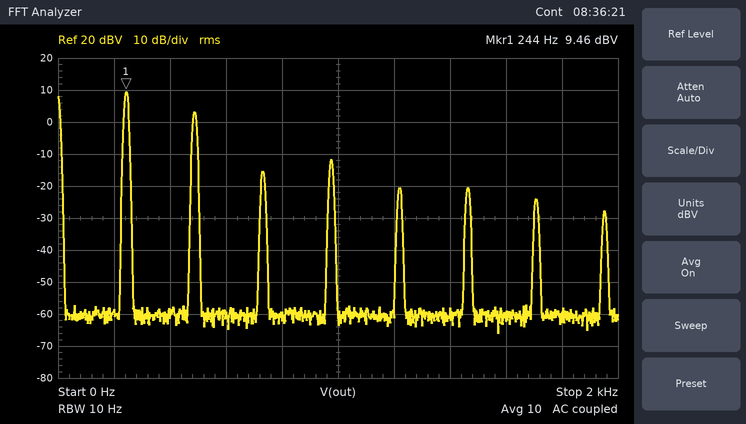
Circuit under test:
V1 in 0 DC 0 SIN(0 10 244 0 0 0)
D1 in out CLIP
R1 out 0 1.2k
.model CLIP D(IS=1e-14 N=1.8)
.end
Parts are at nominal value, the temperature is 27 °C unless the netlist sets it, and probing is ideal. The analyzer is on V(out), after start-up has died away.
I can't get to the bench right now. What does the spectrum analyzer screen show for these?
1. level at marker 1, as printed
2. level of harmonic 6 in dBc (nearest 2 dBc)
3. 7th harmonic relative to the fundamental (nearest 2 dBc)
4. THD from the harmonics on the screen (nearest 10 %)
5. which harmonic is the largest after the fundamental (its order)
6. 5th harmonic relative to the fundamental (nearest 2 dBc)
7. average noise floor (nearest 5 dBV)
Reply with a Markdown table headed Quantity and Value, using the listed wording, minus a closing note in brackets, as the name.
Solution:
| Quantity | Value |
|---|---|
| level at marker 1, as printed | 9.46 dBV |
| level of harmonic 6 in dBc | -30 dBc |
| 7th harmonic relative to the fundamental | -34 dBc |
| THD from the harmonics on the screen | 50 % |
| which harmonic is the largest after the fundamental | 2 |
| 5th harmonic relative to the fundamental | -30 dBc |
| average noise floor | -60 dBV |
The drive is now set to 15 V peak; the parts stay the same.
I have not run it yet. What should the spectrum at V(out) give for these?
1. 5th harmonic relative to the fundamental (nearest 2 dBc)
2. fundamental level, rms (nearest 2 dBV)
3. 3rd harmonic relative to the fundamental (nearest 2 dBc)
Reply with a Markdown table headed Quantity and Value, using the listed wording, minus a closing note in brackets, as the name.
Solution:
| Quantity | Value |
|---|---|
| 5th harmonic relative to the fundamental | -34 dBc |
| fundamental level, rms | 14 dBV |
| 3rd harmonic relative to the fundamental | -28 dBc |
